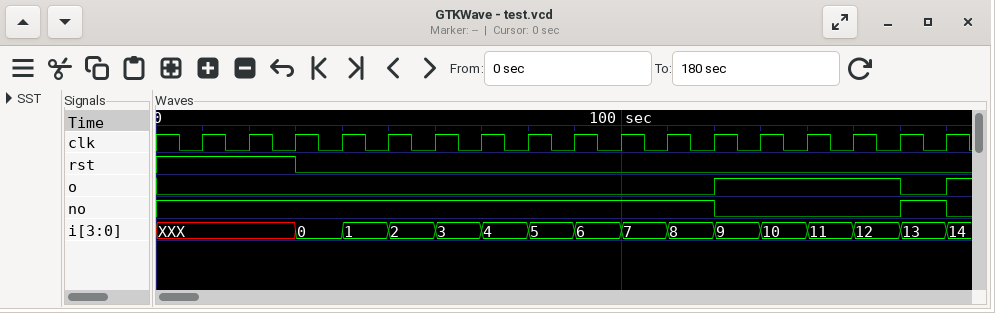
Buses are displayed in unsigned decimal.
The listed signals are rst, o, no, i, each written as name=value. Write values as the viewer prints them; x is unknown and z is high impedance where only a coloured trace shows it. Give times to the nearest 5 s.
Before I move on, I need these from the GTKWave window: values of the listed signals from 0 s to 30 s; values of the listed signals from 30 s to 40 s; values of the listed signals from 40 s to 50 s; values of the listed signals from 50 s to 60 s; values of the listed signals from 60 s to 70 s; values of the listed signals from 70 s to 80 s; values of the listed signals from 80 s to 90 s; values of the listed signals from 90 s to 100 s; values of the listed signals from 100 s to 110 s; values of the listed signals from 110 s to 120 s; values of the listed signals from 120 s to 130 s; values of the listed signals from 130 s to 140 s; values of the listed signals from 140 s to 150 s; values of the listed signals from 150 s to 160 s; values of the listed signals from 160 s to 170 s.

rst=1, o=0, no=1, i=XXX
rst=0, o=0, no=1, i=0
rst=0, o=0, no=1, i=1
rst=0, o=0, no=1, i=2
rst=0, o=0, no=1, i=3
rst=0, o=0, no=1, i=4
rst=0, o=0, no=1, i=5
rst=0, o=0, no=1, i=6
rst=0, o=0, no=1, i=7
rst=0, o=0, no=1, i=8
rst=0, o=1, no=0, i=9
rst=0, o=1, no=0, i=10
rst=0, o=1, no=0, i=11
rst=0, o=1, no=0, i=12
rst=0, o=0, no=1, i=13
